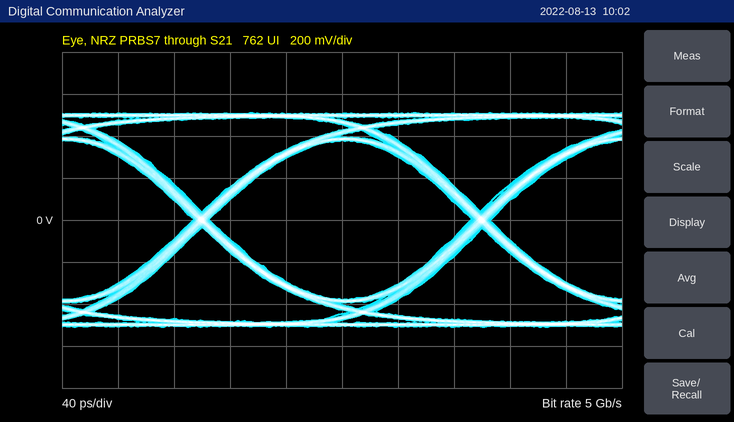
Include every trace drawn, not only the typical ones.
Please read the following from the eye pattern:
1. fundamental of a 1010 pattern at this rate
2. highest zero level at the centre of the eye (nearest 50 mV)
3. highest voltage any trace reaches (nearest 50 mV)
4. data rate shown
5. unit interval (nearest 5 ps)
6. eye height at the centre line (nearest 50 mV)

2.5 GHz
-400 mV
500 mV
5 Gb/s
200 ps
750 mV
